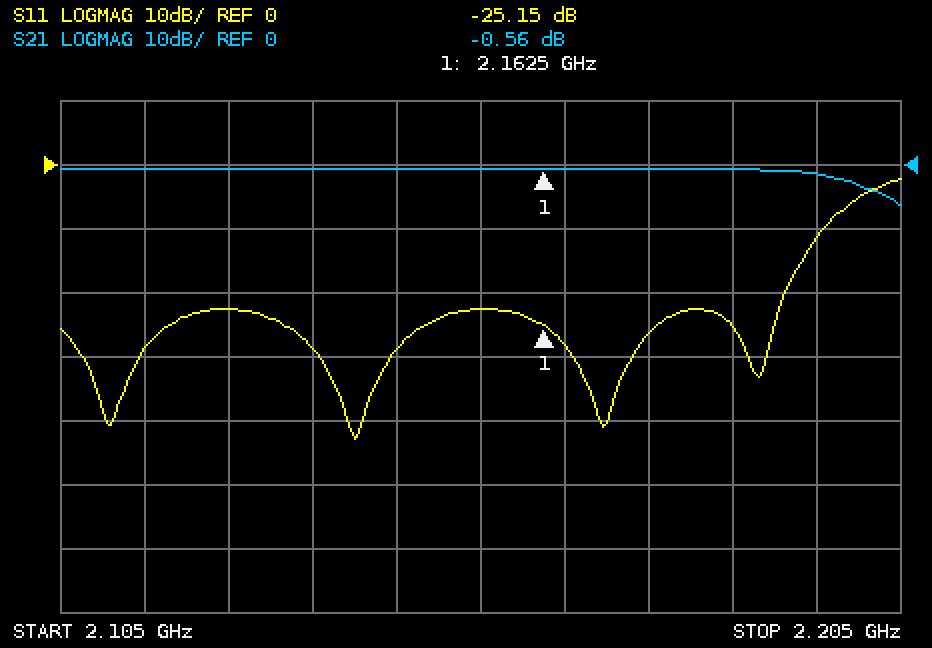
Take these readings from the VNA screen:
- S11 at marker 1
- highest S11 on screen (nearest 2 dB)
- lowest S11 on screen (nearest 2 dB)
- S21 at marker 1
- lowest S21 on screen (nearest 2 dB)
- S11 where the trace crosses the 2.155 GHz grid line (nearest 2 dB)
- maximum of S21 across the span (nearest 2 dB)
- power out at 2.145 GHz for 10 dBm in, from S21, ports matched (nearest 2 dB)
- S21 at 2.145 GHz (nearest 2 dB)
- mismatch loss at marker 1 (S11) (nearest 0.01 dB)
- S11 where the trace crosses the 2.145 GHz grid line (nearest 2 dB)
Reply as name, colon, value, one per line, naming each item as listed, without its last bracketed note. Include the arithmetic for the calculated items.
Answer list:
S11 at marker 1: -25.15 dB
highest S11 on screen: -2 dB
lowest S11 on screen: -42 dB
S21 at marker 1: -0.56 dB
lowest S21 on screen: -6 dB
S11 where the trace crosses the 2.155 GHz grid line: -22 dB
maximum of S21 across the span: 0 dB
power out at 2.145 GHz for 10 dBm in, from S21, ports matched: 10 dBm + (0 dB) = 10 dBm
S21 at 2.145 GHz: 0 dB
mismatch loss at marker 1 (S11): −10 log10(1 − 10^(-25.15/10)) ≈ 0.01 dB
S11 where the trace crosses the 2.145 GHz grid line: -28 dB
